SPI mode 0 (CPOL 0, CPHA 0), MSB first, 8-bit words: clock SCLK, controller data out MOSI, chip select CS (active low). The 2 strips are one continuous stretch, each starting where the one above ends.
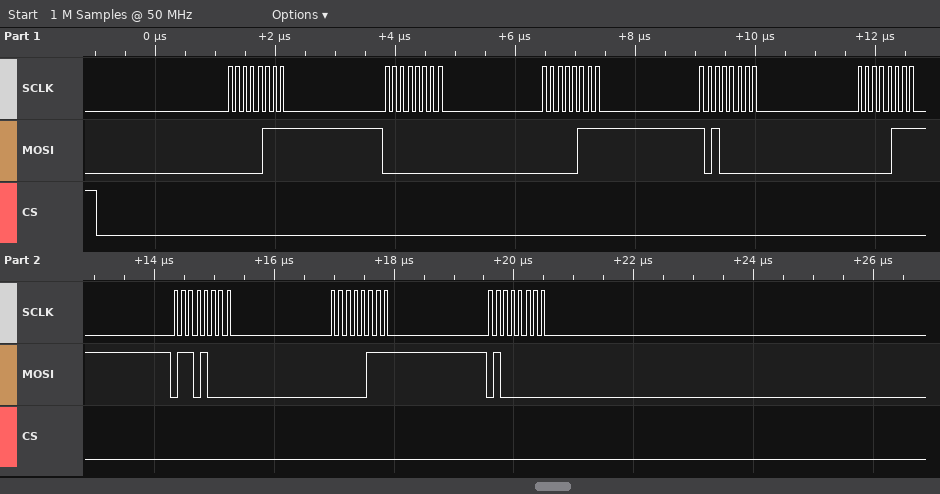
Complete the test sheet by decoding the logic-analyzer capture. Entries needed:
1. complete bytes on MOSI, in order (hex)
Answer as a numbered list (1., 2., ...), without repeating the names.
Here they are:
1. 07 00 07 A0 07 68 07 40
